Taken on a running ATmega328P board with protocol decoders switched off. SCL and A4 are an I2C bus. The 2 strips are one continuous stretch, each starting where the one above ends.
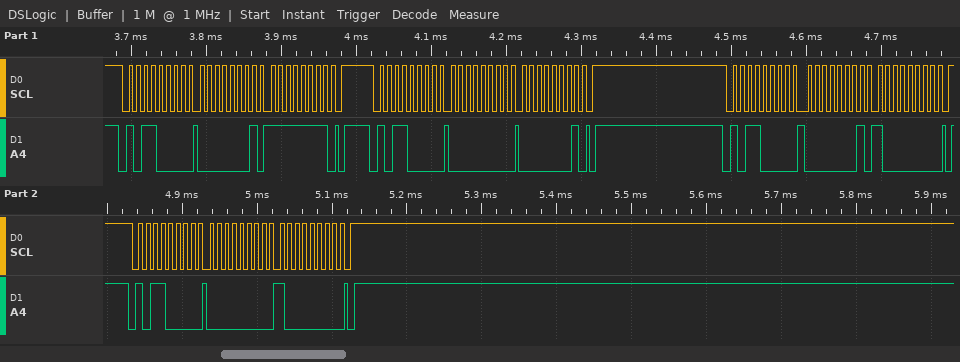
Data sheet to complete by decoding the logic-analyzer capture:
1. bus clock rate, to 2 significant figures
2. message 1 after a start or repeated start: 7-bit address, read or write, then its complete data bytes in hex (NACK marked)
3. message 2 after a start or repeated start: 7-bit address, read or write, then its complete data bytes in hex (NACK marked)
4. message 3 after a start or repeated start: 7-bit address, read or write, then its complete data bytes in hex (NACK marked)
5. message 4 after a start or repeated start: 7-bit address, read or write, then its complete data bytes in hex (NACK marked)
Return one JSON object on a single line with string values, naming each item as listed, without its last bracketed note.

{"bus clock rate, to 2 significant figures": "100 kHz", "message 1 after a start or repeated start: 7-bit address, read or write, then its complete data bytes in hex": "0x58 write: 01 FF", "message 2 after a start or repeated start: 7-bit address, read or write, then its complete data bytes in hex": "0x58 write: 00 01", "message 3 after a start or repeated start: 7-bit address, read or write, then its complete data bytes in hex": "0x58 write: 01 80", "message 4 after a start or repeated start: 7-bit address, read or write, then its complete data bytes in hex": "0x58 write: 00 80"}
